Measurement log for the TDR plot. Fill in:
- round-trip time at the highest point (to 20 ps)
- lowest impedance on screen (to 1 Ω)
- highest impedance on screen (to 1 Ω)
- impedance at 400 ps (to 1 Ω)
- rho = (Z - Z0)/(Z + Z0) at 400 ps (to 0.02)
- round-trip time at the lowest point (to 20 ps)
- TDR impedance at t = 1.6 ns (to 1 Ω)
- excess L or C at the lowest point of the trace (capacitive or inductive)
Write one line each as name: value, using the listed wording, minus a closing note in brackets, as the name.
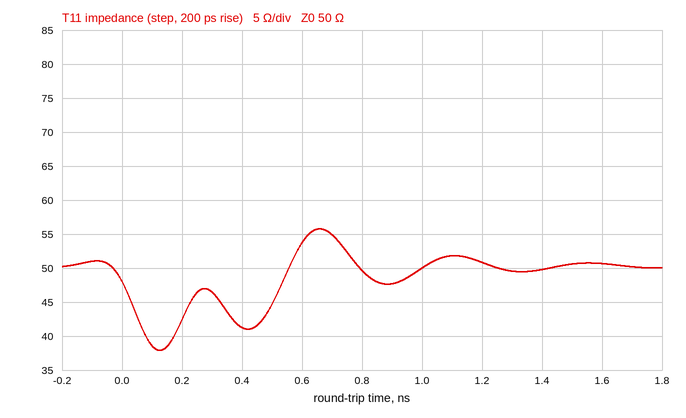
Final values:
round-trip time at the highest point: 660 ps
lowest impedance on screen: 38 Ω
highest impedance on screen: 56 Ω
impedance at 400 ps: 41 Ω
rho = (Z - Z0)/(Z + Z0) at 400 ps: -0.10
round-trip time at the lowest point: 120 ps
TDR impedance at t = 1.6 ns: 51 Ω
excess L or C at the lowest point of the trace: capacitive
